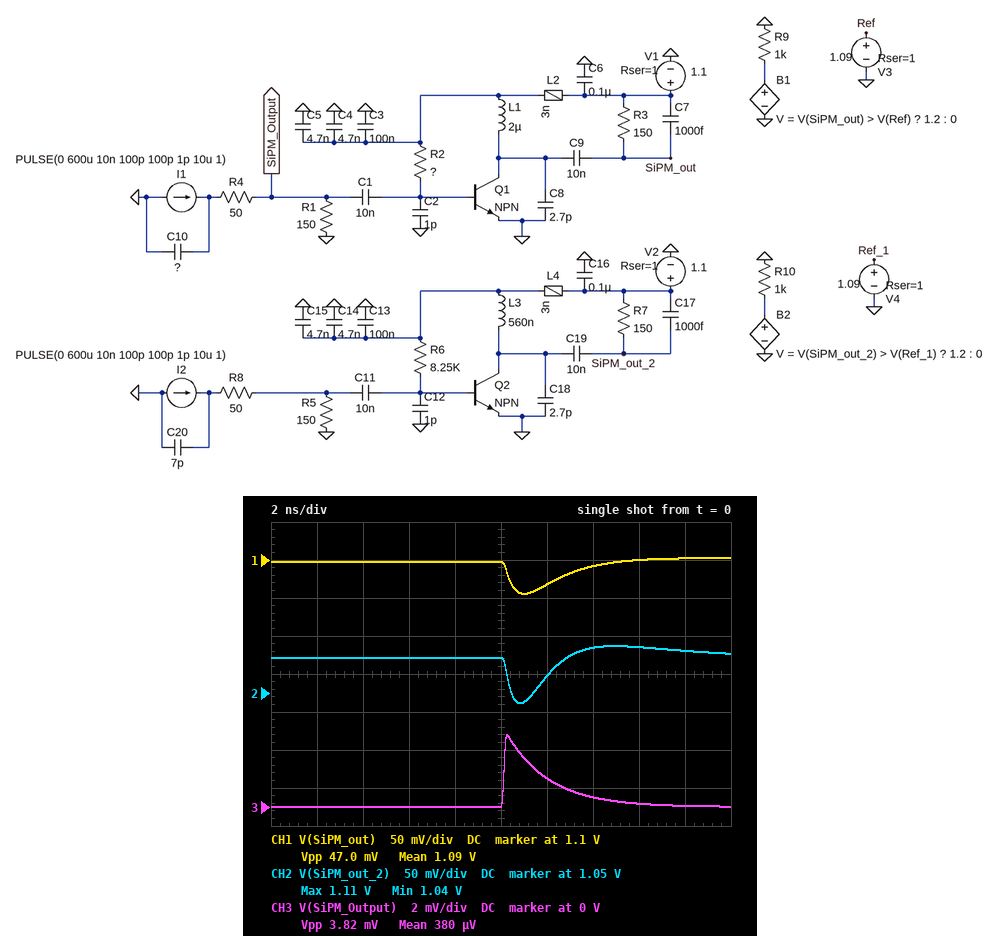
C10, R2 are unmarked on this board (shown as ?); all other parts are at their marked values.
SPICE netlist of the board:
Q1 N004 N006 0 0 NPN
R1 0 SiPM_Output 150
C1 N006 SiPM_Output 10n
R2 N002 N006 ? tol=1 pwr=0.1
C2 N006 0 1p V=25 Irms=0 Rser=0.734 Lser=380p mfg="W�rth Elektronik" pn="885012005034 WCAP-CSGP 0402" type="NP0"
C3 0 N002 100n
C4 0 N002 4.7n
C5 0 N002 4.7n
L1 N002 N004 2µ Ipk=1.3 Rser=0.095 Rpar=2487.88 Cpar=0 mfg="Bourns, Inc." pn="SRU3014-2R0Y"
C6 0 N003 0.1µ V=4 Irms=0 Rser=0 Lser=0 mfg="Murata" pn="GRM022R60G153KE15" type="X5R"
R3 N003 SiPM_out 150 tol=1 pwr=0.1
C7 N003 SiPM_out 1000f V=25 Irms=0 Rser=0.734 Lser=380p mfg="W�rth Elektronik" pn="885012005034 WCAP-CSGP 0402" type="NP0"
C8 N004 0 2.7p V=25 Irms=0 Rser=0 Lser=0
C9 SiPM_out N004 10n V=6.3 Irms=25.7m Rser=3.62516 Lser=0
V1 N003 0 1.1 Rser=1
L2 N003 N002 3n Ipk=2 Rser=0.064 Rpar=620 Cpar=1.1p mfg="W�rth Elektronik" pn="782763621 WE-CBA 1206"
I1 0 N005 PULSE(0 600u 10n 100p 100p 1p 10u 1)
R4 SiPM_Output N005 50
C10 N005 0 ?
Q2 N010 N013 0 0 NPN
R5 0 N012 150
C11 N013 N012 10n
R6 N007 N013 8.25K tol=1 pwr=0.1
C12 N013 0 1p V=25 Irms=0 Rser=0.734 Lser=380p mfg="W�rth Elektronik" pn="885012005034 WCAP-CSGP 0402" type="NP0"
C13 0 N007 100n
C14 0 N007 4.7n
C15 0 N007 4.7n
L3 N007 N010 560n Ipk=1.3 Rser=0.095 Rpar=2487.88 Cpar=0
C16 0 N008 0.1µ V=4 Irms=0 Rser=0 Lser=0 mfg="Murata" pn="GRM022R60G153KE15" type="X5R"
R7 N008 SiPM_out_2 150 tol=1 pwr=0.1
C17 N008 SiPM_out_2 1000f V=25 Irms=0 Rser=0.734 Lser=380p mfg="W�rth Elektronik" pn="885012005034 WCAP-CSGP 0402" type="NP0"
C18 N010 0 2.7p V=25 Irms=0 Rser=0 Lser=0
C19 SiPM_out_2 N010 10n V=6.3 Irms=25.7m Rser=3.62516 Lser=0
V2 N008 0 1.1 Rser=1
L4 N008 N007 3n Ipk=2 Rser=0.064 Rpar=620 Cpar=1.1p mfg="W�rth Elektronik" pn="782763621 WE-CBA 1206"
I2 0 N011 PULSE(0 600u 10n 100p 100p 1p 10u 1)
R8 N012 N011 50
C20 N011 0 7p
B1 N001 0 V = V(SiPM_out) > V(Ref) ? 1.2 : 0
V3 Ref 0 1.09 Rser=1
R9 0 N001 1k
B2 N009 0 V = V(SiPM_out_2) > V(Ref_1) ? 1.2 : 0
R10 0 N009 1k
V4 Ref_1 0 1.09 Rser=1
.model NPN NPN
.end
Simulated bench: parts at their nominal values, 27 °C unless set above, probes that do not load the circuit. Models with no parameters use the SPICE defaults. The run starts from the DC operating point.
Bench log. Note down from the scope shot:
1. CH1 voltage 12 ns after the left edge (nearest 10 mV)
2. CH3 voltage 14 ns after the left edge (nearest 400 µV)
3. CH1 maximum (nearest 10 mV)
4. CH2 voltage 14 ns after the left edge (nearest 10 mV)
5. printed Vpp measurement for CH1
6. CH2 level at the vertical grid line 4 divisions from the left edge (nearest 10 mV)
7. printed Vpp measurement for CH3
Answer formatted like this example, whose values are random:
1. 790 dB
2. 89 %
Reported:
1. 1.07 V
2. 400 µV
3. 1.10 V
4. 1.11 V
5. 47.0 mV
6. 1.10 V
7. 3.82 mV
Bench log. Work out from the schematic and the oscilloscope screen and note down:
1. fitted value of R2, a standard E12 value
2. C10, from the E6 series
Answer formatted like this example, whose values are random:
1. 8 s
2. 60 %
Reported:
1. 10 kΩ
2. 10 pF
